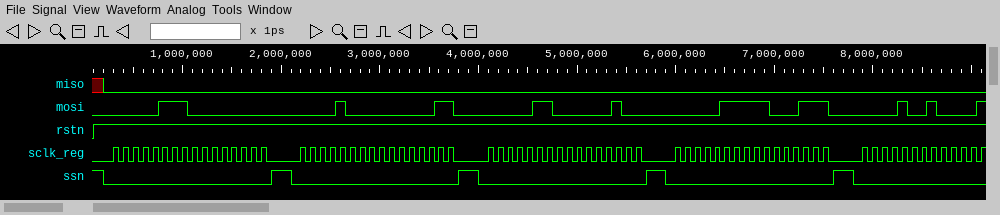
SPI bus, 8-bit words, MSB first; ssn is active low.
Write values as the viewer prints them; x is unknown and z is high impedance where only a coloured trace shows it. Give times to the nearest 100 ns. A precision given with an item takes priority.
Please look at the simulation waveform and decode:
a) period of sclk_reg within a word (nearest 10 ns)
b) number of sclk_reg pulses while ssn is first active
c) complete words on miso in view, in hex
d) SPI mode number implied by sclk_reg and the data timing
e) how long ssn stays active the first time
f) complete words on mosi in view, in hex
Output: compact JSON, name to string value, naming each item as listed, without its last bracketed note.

{"period of sclk_reg within a word": "100 ns", "number of sclk_reg pulses while ssn is first active": "16", "complete words on miso in view, in hex": "00, 00, 00, 00, 00, 00, 00, 00, 00", "SPI mode number implied by sclk_reg and the data timing": "0", "how long ssn stays active the first time": "1700 ns", "complete words on mosi in view, in hex": "07, 00, 08, 03, 06, 04, 07, C7, 09"}
